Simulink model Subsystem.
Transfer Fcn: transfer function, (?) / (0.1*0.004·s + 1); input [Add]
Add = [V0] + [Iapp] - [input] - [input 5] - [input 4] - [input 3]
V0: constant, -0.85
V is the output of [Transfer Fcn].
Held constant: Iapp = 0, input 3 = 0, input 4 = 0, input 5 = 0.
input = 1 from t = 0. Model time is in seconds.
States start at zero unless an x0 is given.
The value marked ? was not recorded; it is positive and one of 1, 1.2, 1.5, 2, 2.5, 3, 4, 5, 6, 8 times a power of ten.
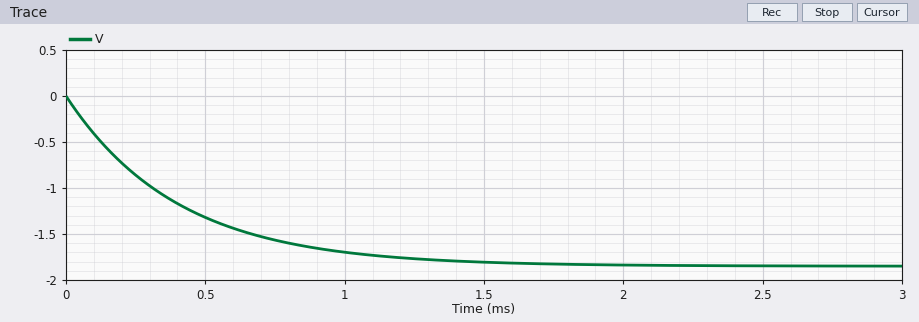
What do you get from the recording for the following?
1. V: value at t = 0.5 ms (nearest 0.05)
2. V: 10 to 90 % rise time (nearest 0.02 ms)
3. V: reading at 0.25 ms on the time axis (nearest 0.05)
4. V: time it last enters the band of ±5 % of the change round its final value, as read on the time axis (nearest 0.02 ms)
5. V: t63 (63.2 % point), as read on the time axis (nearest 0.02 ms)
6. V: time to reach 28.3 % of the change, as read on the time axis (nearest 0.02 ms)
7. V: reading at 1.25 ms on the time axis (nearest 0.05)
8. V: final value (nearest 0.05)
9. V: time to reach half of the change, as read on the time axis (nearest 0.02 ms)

-1.30
0.88 ms
-0.85
1.20 ms
0.40 ms
0.14 ms
-1.75
-1.85
0.28 ms
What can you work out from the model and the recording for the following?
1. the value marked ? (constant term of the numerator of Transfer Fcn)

1
